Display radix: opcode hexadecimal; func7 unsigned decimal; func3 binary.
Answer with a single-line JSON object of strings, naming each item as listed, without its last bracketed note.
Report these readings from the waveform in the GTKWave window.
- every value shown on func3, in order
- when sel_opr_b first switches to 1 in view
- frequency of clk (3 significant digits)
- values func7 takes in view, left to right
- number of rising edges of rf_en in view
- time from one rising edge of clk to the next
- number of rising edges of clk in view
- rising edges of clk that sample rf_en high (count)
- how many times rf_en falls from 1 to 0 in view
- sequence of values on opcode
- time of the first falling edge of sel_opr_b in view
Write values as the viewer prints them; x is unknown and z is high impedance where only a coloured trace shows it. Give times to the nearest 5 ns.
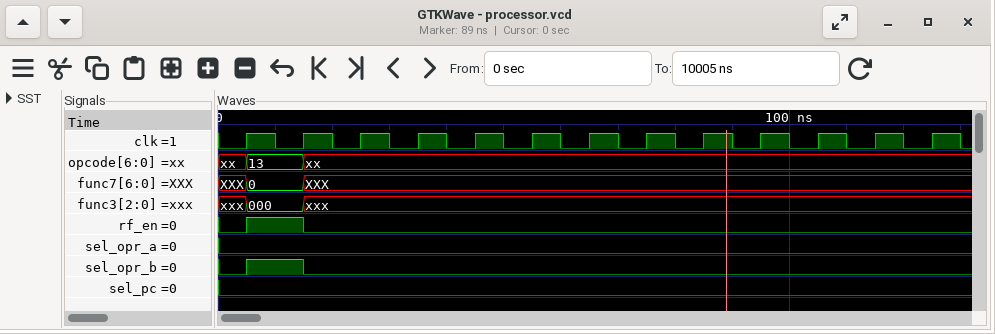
{"every value shown on func3, in order": "xxx, 000, xxx", "when sel_opr_b first switches to 1 in view": "5 ns", "frequency of clk": "100 MHz", "values func7 takes in view, left to right": "XXX, 0, XXX", "number of rising edges of rf_en in view": "1", "time from one rising edge of clk to the next": "10 ns", "number of rising edges of clk in view": "13", "rising edges of clk that sample rf_en high": "1", "how many times rf_en falls from 1 to 0 in view": "1", "sequence of values on opcode": "xx, 13, xx", "time of the first falling edge of sel_opr_b in view": "15 ns"}
